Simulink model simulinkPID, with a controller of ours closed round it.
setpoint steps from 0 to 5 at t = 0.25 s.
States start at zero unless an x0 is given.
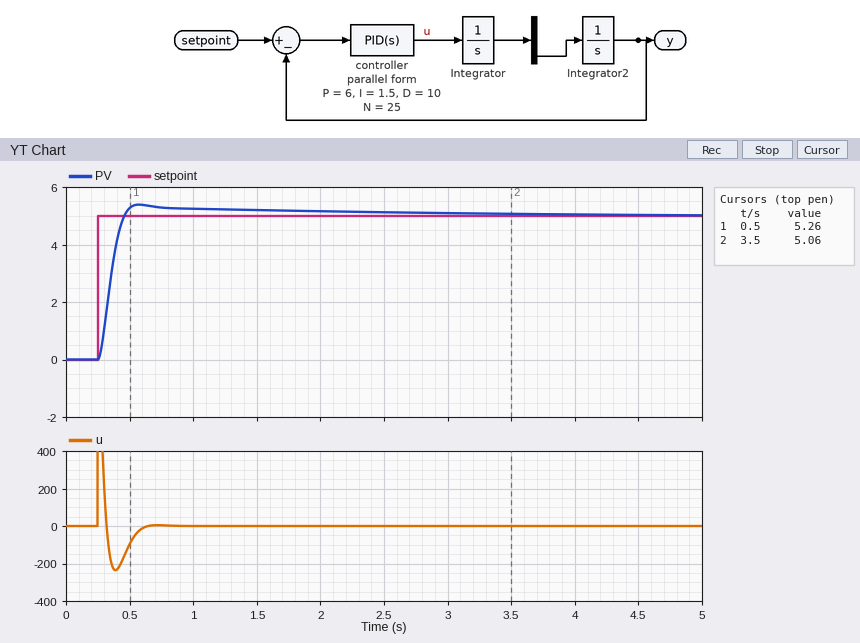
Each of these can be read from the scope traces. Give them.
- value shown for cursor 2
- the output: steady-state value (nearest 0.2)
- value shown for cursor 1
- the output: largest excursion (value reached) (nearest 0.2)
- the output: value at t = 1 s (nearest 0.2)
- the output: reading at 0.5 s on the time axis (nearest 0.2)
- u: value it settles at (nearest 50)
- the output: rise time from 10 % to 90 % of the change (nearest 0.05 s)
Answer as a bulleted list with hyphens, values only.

- 5.06
- 5.0
- 5.26
- 5.4
- 5.2
- 5.2
- 0
- 0.15 s
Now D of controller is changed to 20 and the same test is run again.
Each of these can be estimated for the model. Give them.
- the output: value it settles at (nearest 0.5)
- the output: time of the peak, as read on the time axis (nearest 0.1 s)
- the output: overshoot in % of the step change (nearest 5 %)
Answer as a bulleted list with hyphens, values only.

- 5.0
- 0.4 s
- 15 %
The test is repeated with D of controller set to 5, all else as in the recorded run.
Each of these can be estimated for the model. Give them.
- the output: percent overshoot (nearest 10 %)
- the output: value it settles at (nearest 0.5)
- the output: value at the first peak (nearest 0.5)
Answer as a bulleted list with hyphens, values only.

- 20 %
- 5.0
- 6.0
